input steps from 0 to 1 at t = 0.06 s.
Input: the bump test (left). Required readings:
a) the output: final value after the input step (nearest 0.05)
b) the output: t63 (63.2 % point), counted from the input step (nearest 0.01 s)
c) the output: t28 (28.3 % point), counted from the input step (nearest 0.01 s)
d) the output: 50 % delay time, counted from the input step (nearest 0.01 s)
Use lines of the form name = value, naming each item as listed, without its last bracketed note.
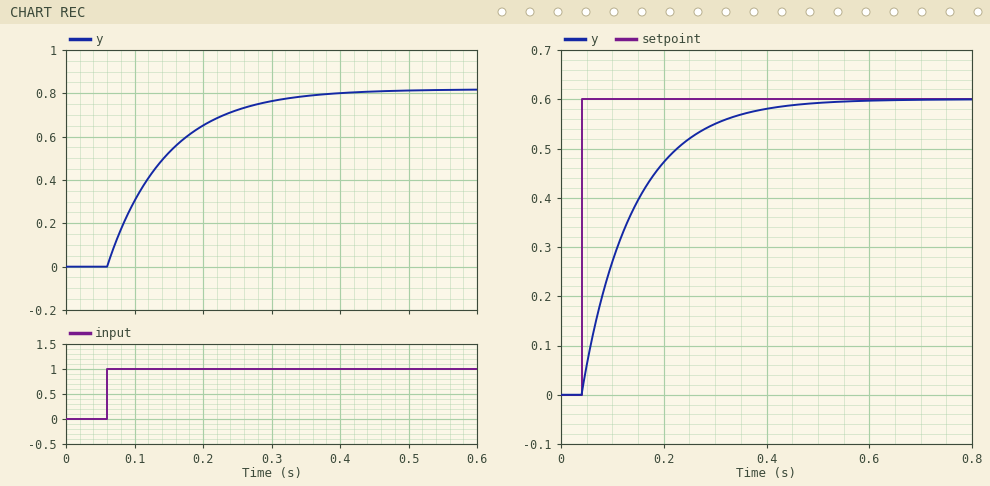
the output: final value after the input step = 0.80
the output: t63 (63.2 % point), counted from the input step = 0.09 s
the output: t28 (28.3 % point), counted from the input step = 0.03 s
the output: 50 % delay time, counted from the input step = 0.06 s
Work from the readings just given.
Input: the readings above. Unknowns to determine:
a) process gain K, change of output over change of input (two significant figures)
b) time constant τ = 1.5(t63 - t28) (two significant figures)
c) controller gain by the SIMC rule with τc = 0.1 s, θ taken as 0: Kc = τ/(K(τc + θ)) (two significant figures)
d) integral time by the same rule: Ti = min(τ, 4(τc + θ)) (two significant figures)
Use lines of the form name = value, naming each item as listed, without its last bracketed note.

process gain K, change of output over change of input = 0.80
time constant τ = 1.5(t63 - t28) = 0.090 s
controller gain by the SIMC rule with τc = 0.1 s, θ taken as 0: Kc = τ/(K(τc + θ)) = 1.1
integral time by the same rule: Ti = min(τ, 4(τc + θ)) = 0.090 s
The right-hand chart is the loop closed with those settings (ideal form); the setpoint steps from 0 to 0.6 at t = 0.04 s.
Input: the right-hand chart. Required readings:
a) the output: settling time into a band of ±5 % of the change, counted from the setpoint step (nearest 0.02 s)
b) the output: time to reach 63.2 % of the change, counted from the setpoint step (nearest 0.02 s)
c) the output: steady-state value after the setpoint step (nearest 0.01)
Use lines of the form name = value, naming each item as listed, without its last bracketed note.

the output: settling time into a band of ±5 % of the change, counted from the setpoint step = 0.32 s
the output: time to reach 63.2 % of the change, counted from the setpoint step = 0.10 s
the output: steady-state value after the setpoint step = 0.60
